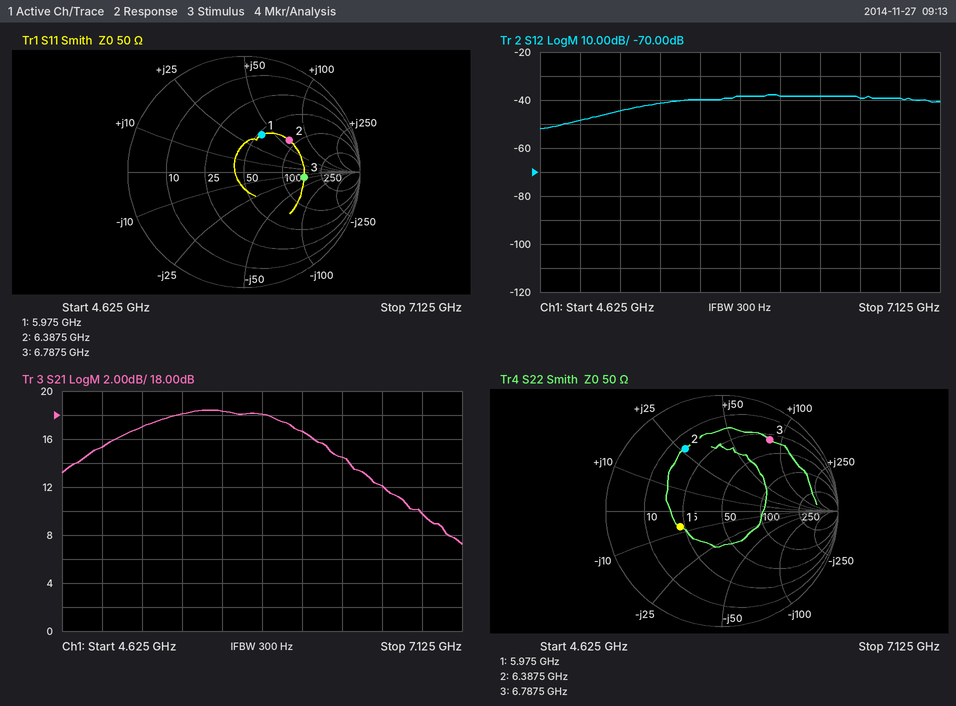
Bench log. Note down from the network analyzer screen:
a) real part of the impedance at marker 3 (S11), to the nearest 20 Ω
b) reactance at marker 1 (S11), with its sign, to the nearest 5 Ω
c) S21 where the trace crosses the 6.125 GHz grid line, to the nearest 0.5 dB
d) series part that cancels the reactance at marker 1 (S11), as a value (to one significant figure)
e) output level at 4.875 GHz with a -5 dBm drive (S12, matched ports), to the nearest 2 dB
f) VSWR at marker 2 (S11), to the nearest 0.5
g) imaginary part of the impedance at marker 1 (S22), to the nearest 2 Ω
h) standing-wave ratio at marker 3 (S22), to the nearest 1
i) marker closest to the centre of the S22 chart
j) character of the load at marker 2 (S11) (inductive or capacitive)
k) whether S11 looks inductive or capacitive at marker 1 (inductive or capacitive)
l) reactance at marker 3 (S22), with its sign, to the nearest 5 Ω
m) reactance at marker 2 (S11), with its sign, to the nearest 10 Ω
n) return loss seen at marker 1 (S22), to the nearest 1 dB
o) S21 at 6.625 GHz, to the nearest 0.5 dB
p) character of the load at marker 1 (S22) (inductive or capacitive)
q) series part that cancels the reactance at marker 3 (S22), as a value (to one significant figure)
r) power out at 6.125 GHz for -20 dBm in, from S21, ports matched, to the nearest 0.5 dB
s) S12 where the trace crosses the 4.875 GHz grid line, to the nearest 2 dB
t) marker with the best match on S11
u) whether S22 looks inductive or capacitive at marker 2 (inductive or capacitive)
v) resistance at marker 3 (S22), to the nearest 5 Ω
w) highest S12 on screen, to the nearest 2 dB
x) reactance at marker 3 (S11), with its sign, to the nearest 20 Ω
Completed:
160 Ω
+40 Ω
16.5 dB
700 fF
-54 dBm
3.0
-8 Ω
7
marker 1
inductive
inductive
+85 Ω
+60 Ω
8 dB
12.0 dB
capacitive
300 fF
-3.5 dBm
-48 dB
marker 1
inductive
30 Ω
-38 dB
-20 Ω
